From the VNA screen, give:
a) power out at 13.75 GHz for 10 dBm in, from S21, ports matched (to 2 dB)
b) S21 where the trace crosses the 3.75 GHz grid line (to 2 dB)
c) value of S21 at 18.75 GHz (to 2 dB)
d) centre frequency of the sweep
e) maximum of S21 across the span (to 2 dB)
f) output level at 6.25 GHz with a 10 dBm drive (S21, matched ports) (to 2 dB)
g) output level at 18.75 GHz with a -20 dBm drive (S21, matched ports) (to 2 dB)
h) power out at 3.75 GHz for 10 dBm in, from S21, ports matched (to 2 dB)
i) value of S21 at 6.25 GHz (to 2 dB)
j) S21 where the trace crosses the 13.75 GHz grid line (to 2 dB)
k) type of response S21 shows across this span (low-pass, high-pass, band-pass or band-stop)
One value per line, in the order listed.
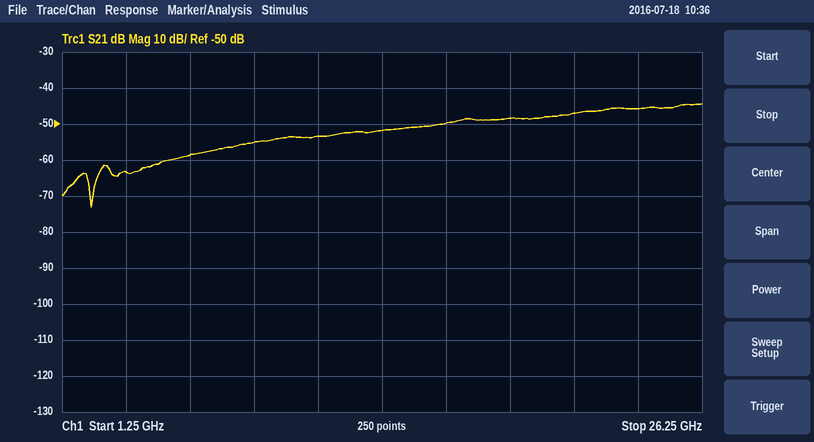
-42 dBm
-64 dB
-48 dB
13.75 GHz
-44 dB
-48 dBm
-68 dBm
-54 dBm
-58 dB
-52 dB
high-pass
